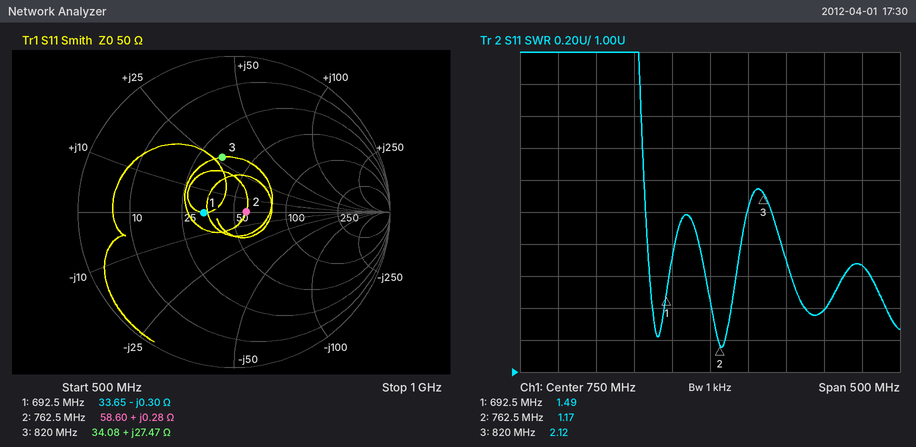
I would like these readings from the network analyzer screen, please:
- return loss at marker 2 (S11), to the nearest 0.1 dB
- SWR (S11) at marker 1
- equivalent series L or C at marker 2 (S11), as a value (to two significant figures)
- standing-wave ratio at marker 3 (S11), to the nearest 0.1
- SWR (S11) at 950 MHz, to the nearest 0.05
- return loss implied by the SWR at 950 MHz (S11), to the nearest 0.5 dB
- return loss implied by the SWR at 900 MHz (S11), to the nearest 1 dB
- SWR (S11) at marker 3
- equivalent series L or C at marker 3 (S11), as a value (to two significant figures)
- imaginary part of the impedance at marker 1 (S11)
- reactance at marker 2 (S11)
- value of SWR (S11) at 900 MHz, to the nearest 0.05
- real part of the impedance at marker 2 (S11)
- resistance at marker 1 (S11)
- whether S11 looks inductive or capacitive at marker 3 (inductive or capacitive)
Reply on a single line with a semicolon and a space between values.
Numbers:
22.0 dB; 1.49; 58 pH; 2.1; 1.65; 12.0 dB; 16 dB; 2.12; 5.3 nH; -0.30 Ω; +0.28 Ω; 1.40; 58.60 Ω; 33.65 Ω; inductive
